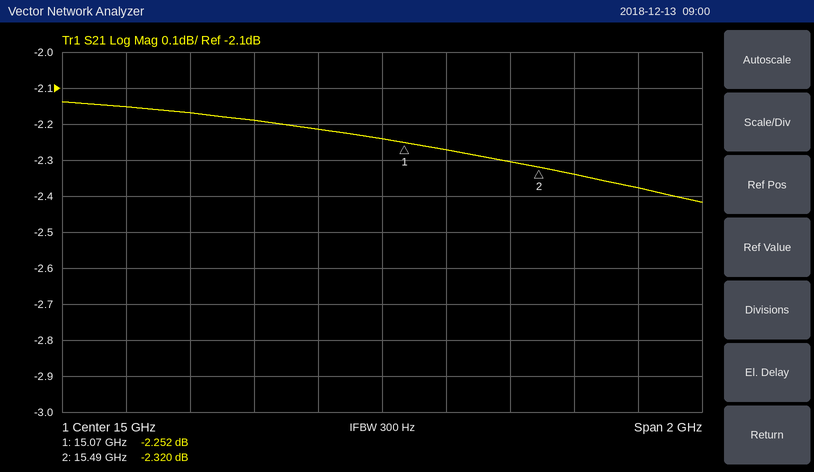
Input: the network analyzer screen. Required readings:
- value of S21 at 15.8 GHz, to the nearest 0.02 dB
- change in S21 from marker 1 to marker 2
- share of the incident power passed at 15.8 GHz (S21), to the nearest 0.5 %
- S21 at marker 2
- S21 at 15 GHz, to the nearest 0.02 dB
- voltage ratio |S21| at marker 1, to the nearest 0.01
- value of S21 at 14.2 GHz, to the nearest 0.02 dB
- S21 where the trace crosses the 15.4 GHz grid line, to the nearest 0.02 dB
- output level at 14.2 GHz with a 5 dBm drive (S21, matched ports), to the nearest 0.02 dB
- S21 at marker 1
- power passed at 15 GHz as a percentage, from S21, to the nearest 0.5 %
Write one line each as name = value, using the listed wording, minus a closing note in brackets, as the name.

value of S21 at 15.8 GHz, to the nearest 0.02 dB = -2.38 dB
change in S21 from marker 1 to marker 2 = -0.068 dB
share of the incident power passed at 15.8 GHz (S21), to the nearest 0.5 % = 58.0 %
S21 at marker 2 = -2.320 dB
S21 at 15 GHz, to the nearest 0.02 dB = -2.24 dB
voltage ratio |S21| at marker 1, to the nearest 0.01 = 0.77
value of S21 at 14.2 GHz, to the nearest 0.02 dB = -2.16 dB
S21 where the trace crosses the 15.4 GHz grid line, to the nearest 0.02 dB = -2.30 dB
output level at 14.2 GHz with a 5 dBm drive (S21, matched ports), to the nearest 0.02 dB = 2.84 dBm
S21 at marker 1 = -2.252 dB
power passed at 15 GHz as a percentage, from S21, to the nearest 0.5 % = 59.5 %
